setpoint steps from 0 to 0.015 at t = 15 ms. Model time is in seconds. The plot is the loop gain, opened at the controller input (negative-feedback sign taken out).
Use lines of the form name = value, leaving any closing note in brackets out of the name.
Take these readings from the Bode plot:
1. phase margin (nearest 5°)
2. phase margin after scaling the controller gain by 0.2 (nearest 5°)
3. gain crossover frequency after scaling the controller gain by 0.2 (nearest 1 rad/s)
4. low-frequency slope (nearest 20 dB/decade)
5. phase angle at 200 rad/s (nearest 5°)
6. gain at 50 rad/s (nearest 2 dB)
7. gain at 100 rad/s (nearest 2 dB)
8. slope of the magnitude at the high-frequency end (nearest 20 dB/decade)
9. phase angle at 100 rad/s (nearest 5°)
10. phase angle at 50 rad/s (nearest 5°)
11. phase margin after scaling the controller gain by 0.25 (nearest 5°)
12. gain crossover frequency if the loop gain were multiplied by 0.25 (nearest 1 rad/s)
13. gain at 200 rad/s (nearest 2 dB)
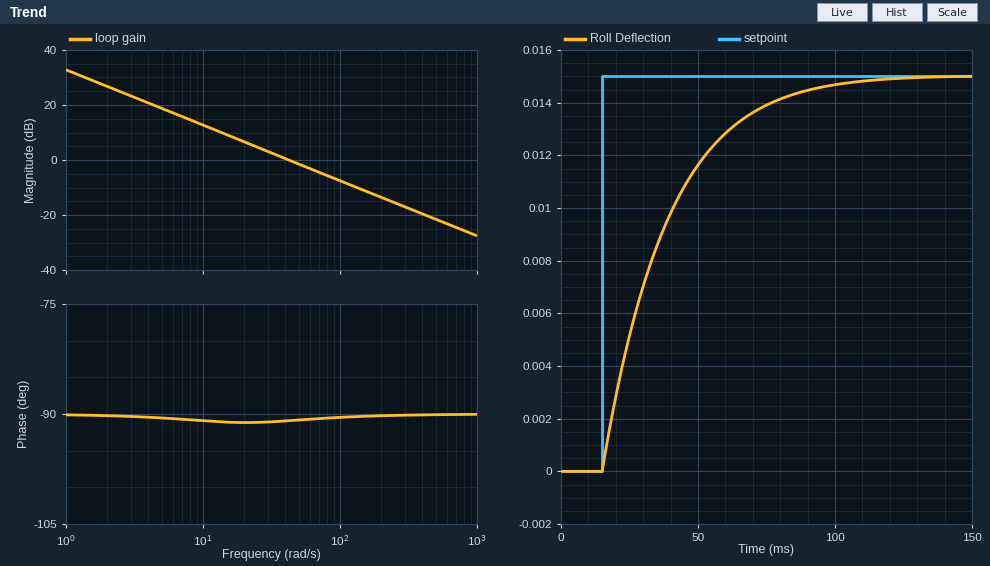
phase margin = 90°
phase margin after scaling the controller gain by 0.2 = 90°
gain crossover frequency after scaling the controller gain by 0.2 = 9 rad/s
low-frequency slope = -20 dB/decade
phase angle at 200 rad/s = -90°
gain at 50 rad/s = -2 dB
gain at 100 rad/s = -8 dB
slope of the magnitude at the high-frequency end = -20 dB/decade
phase angle at 100 rad/s = -90°
phase angle at 50 rad/s = -90°
phase margin after scaling the controller gain by 0.25 = 90°
gain crossover frequency if the loop gain were multiplied by 0.25 = 11 rad/s
gain at 200 rad/s = -14 dB
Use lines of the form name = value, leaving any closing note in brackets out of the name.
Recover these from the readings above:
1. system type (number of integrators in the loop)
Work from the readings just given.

system type = 1
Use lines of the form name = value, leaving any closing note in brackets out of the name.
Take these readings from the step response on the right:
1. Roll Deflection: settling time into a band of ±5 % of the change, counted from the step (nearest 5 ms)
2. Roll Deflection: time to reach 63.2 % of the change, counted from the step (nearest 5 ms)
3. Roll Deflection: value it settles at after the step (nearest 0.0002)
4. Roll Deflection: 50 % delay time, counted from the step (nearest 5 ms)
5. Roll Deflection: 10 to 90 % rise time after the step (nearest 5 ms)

Roll Deflection: settling time into a band of ±5 % of the change, counted from the step = 70 ms
Roll Deflection: time to reach 63.2 % of the change, counted from the step = 25 ms
Roll Deflection: value it settles at after the step = 0.0150
Roll Deflection: 50 % delay time, counted from the step = 15 ms
Roll Deflection: 10 to 90 % rise time after the step = 50 ms
